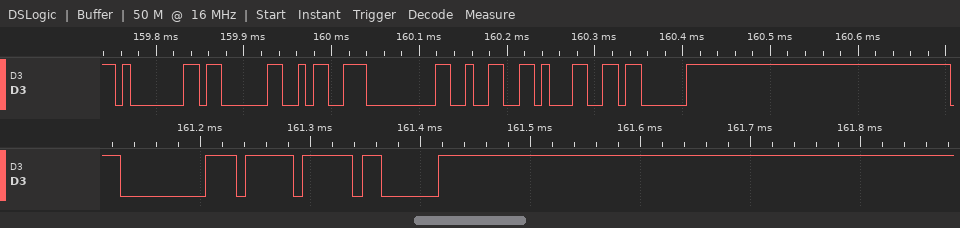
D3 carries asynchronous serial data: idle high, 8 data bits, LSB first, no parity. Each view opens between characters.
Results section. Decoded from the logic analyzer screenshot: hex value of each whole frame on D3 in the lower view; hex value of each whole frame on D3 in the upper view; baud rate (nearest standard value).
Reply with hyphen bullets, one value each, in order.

- 00, DF, 03
- 01, 03, 9A, 00, 32, 31, 03
- 115200 baud
